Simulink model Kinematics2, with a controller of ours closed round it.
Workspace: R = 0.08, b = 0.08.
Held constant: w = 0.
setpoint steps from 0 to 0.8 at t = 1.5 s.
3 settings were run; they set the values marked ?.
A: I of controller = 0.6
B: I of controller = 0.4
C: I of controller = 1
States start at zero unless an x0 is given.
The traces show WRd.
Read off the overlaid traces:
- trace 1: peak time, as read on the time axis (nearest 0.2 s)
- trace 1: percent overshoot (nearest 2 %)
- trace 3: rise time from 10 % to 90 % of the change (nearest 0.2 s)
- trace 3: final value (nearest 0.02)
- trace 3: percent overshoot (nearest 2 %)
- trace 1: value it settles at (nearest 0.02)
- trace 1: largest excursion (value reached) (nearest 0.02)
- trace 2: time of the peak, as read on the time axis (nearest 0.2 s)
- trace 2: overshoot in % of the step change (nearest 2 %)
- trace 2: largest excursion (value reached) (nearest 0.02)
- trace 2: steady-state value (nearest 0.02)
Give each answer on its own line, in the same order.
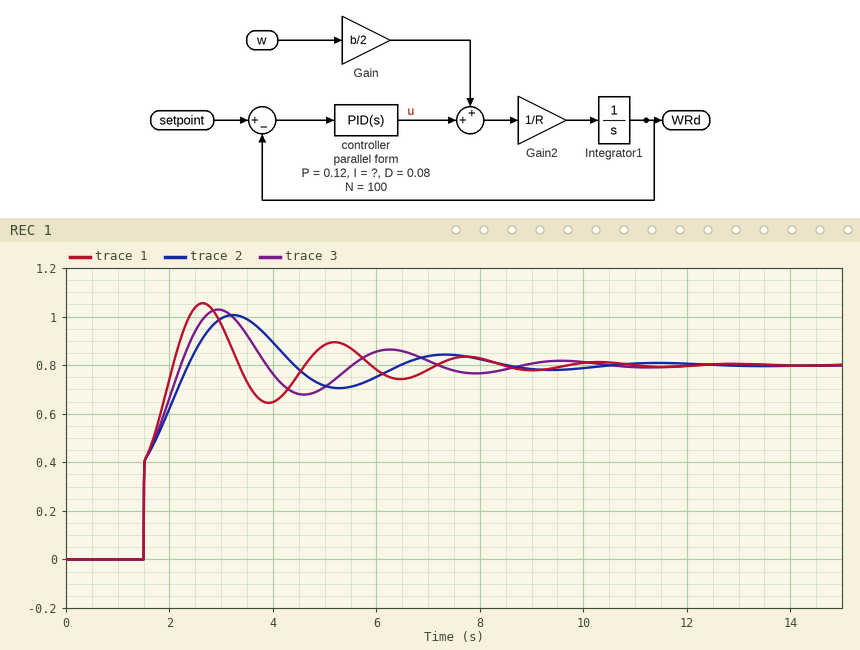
2.6 s
32 %
0.6 s
0.80
28 %
0.80
1.06
3.2 s
26 %
1.00
0.80
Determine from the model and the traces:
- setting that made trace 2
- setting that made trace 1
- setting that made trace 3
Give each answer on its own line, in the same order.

B
C
A
